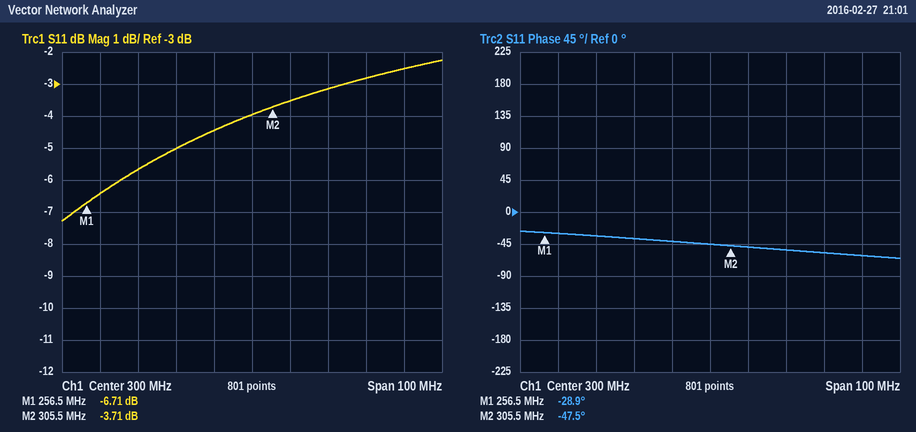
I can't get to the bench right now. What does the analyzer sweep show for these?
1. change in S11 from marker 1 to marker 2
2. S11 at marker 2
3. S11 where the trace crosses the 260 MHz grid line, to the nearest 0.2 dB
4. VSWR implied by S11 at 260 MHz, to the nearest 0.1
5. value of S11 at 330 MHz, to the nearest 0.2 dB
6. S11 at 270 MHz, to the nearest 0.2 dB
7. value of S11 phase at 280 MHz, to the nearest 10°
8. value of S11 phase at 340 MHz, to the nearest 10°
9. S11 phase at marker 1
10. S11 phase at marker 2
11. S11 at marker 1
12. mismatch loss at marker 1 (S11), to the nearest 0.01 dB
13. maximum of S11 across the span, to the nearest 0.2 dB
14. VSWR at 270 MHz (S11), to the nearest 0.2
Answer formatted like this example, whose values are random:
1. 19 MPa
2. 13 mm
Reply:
1. 3.00 dB
2. -3.71 dB
3. -6.4 dB
4. 2.8
5. -2.8 dB
6. -5.6 dB
7. -40°
8. -60°
9. -28.9°
10. -47.5°
11. -6.71 dB
12. 1.04 dB
13. -2.2 dB
14. 3.2
